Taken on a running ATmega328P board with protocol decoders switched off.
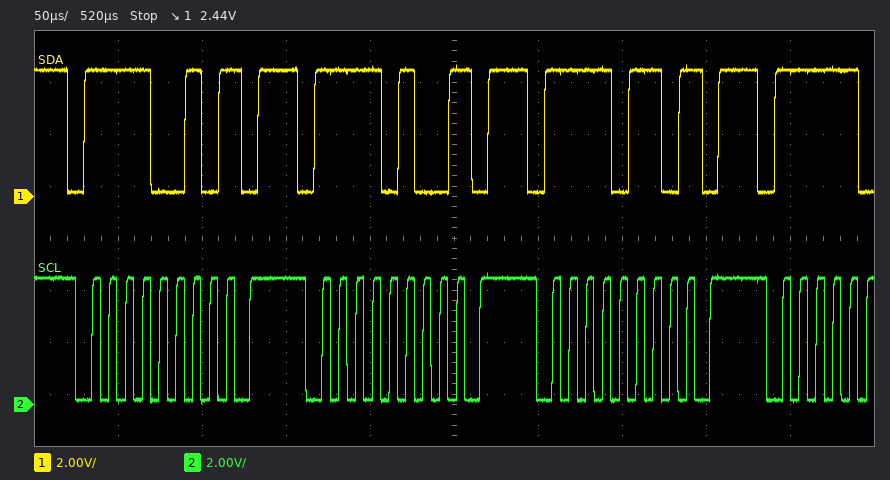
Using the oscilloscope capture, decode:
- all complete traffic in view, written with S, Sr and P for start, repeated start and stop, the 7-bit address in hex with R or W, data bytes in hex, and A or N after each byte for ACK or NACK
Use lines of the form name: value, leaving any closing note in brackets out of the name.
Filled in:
all complete traffic in view, written with S, Sr and P for start, repeated start and stop, the 7-bit address in hex with R or W, data bytes in hex, and A or N after each byte for ACK or NACK: S 79W N P S 7AW N P S 7BW N P
